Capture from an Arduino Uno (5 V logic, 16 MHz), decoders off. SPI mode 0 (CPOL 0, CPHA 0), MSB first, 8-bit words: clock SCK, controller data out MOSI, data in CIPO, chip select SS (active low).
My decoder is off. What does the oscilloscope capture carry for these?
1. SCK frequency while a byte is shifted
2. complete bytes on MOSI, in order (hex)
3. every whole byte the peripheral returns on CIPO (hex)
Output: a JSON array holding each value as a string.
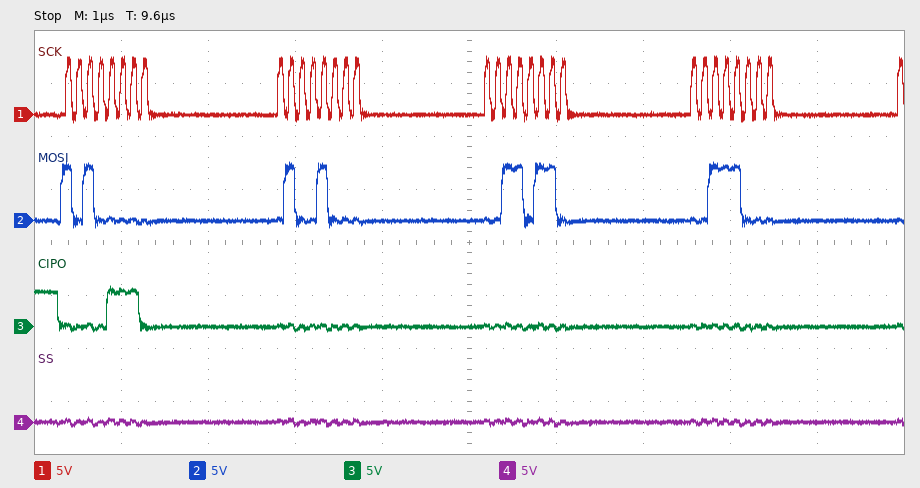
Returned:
["8 MHz", "0xA0 0x48 0x36 0x38", "0x0E 0x00 0x00 0x00"]
